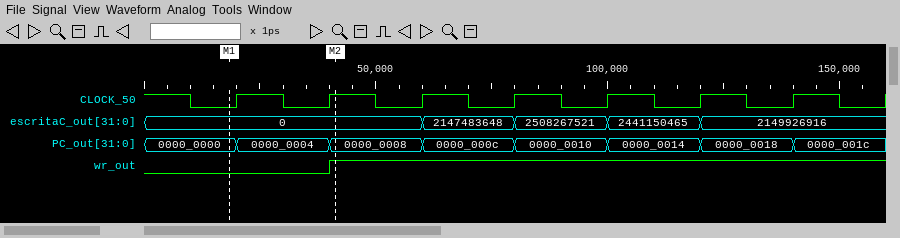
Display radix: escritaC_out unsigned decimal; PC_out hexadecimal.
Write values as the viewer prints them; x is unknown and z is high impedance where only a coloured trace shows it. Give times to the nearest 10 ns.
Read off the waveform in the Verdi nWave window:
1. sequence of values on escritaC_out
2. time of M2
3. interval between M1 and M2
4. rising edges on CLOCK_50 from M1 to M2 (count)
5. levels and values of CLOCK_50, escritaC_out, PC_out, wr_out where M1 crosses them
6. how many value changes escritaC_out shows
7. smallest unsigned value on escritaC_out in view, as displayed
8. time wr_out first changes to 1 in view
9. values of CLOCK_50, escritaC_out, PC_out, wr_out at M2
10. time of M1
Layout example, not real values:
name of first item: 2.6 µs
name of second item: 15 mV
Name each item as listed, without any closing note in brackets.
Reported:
sequence of values on escritaC_out: 0, 2147483648, 2508267521, 2441150465, 2149926916
time of M2: 40 ns
interval between M1 and M2: 20 ns
rising edges on CLOCK_50 from M1 to M2: 2
levels and values of CLOCK_50, escritaC_out, PC_out, wr_out where M1 crosses them: CLOCK_50=0, escritaC_out=0, PC_out=0000_0000, wr_out=0
how many value changes escritaC_out shows: 4
smallest unsigned value on escritaC_out in view, as displayed: 0
time wr_out first changes to 1 in view: 40 ns
values of CLOCK_50, escritaC_out, PC_out, wr_out at M2: CLOCK_50=1, escritaC_out=0, PC_out=0000_0008, wr_out=1
time of M1: 20 ns
